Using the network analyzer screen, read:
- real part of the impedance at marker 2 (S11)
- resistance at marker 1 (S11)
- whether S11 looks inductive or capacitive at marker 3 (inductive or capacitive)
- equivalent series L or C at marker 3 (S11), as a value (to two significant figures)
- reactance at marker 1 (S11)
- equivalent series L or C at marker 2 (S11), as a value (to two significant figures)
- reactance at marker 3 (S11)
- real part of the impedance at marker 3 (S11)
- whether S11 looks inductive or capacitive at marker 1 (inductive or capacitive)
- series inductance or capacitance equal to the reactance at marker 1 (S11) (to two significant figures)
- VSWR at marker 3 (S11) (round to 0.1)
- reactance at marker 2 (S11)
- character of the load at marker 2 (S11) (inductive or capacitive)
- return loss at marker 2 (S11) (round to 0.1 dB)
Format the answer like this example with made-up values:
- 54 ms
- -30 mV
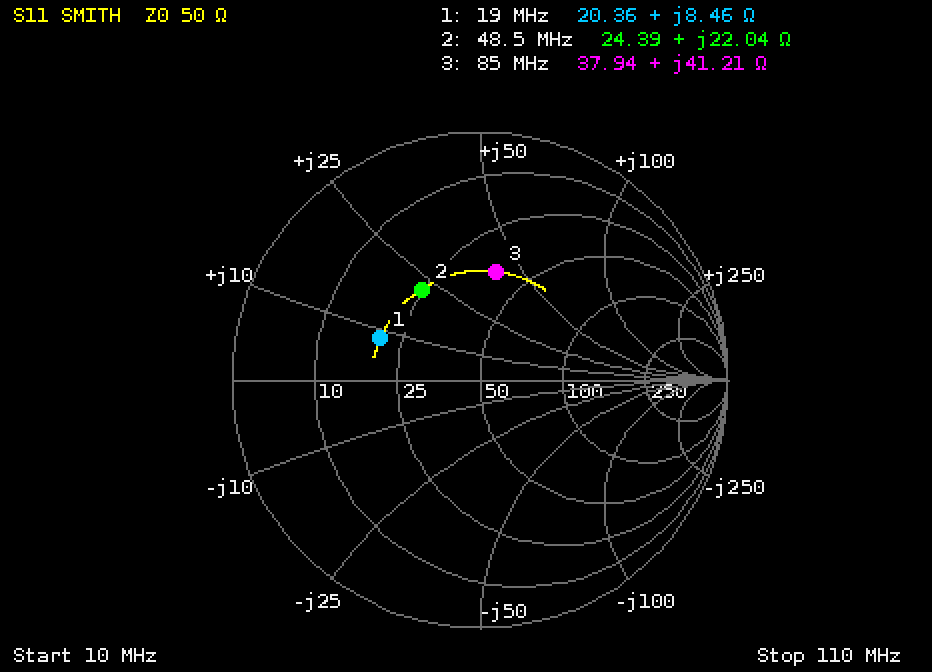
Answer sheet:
- 24.39 Ω
- 20.36 Ω
- inductive
- 77 nH
- +8.46 Ω
- 72 nH
- +41.21 Ω
- 37.94 Ω
- inductive
- 71 nH
- 2.6
- +22.04 Ω
- inductive
- 7.2 dB
